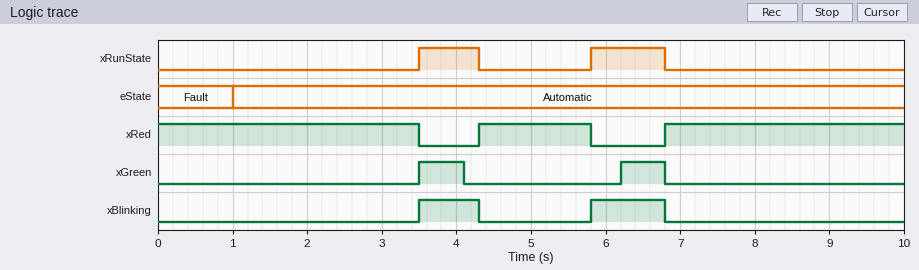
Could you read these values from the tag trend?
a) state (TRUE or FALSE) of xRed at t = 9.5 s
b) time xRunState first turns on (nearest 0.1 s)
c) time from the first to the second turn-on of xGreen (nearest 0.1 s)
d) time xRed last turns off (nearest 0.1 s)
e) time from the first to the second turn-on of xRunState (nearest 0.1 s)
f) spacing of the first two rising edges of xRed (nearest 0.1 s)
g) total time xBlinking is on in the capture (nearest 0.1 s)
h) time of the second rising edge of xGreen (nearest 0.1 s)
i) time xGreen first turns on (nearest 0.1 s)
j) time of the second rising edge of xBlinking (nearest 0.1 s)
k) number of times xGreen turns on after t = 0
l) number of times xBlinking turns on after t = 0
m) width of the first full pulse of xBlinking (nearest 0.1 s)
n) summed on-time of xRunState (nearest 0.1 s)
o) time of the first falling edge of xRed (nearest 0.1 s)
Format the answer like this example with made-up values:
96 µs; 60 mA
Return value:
TRUE; 3.5 s; 2.7 s; 5.8 s; 2.3 s; 2.5 s; 1.8 s; 6.2 s; 3.5 s; 5.8 s; 2; 2; 0.8 s; 1.8 s; 3.5 s
